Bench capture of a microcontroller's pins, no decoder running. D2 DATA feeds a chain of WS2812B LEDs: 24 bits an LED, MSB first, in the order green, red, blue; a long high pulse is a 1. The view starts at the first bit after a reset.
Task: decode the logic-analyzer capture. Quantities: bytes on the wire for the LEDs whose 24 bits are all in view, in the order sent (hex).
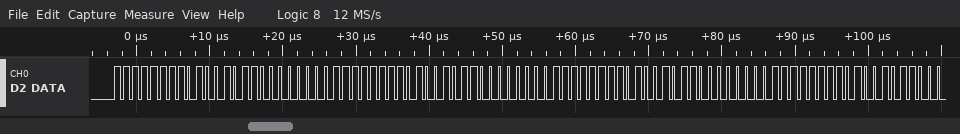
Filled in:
FF 4B 00 FF 4B 00 FF 4B 00
